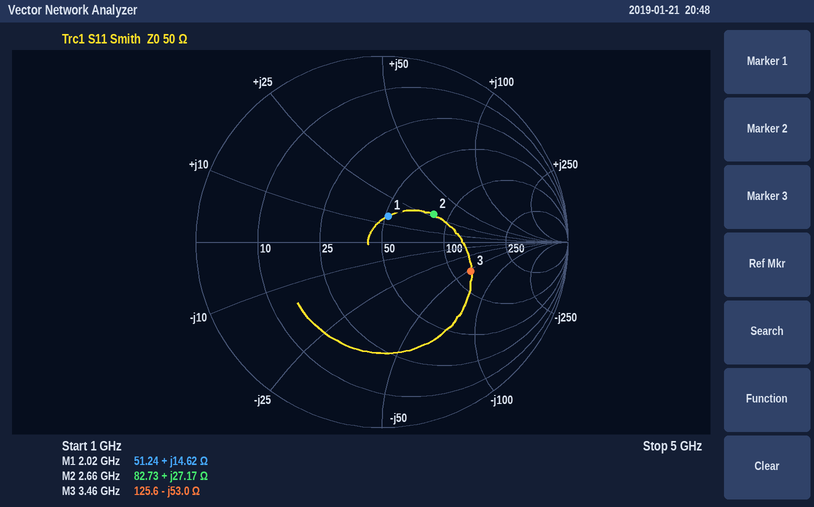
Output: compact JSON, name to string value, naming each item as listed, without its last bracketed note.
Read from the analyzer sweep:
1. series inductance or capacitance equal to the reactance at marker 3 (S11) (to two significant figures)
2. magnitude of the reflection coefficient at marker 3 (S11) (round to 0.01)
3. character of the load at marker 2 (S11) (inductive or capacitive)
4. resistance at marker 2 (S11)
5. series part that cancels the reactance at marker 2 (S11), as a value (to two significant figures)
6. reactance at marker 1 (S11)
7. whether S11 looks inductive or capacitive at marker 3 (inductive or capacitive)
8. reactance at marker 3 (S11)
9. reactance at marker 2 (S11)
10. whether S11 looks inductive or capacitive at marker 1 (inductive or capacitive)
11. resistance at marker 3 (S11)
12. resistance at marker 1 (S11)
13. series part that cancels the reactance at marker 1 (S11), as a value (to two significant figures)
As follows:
{"series inductance or capacitance equal to the reactance at marker 3 (S11)": "870 fF", "magnitude of the reflection coefficient at marker 3 (S11)": "0.50", "character of the load at marker 2 (S11)": "inductive", "resistance at marker 2": "82.73 Ω", "series part that cancels the reactance at marker 2 (S11), as a value": "2.2 pF", "reactance at marker 1": "+14.62 Ω", "whether S11 looks inductive or capacitive at marker 3": "capacitive", "reactance at marker 3": "-53.0 Ω", "reactance at marker 2": "+27.17 Ω", "whether S11 looks inductive or capacitive at marker 1": "inductive", "resistance at marker 3": "125.6 Ω", "resistance at marker 1": "51.24 Ω", "series part that cancels the reactance at marker 1 (S11), as a value": "5.4 pF"}
